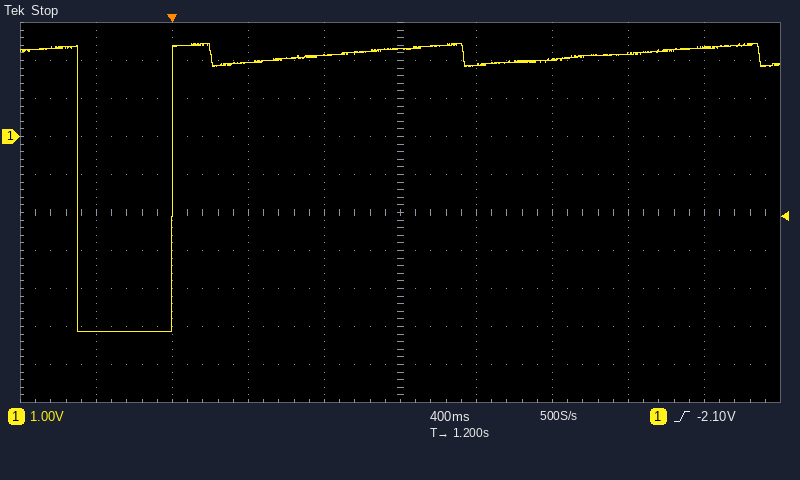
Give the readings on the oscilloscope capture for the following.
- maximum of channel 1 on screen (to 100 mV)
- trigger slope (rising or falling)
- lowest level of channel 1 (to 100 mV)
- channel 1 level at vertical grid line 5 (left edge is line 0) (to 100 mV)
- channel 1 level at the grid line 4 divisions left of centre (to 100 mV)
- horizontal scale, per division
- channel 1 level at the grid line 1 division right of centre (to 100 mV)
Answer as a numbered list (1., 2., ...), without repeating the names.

1. 2.4 V
2. rising
3. -5.1 V
4. 2.3 V
5. -5.1 V
6. 400 ms
7. 1.9 V
